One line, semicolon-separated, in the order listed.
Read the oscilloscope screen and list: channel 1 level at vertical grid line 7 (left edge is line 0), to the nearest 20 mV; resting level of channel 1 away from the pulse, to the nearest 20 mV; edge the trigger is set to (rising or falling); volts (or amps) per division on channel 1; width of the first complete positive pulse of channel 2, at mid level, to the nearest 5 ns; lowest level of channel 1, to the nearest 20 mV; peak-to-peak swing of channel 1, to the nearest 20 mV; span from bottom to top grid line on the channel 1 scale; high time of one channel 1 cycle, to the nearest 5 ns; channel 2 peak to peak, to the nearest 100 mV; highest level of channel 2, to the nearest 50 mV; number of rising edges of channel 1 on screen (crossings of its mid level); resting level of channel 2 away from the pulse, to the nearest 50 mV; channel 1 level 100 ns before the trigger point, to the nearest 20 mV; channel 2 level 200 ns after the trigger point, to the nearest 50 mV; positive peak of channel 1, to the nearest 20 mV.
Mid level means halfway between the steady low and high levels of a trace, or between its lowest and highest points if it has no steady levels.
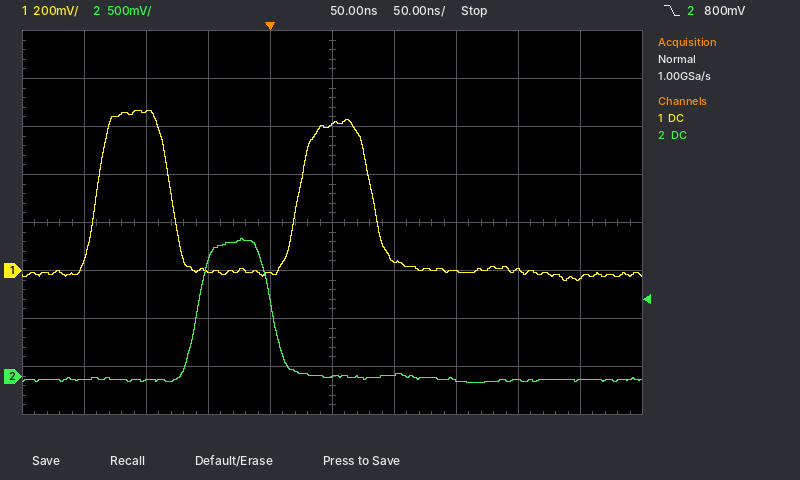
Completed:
0 mV; 0 mV; falling; 200 mV; 60 ns; -40 mV; 700 mV; 1.6 V; 60 ns; 1.50 V; 1.45 V; 2; -50 mV; 660 mV; -50 mV; 660 mV
